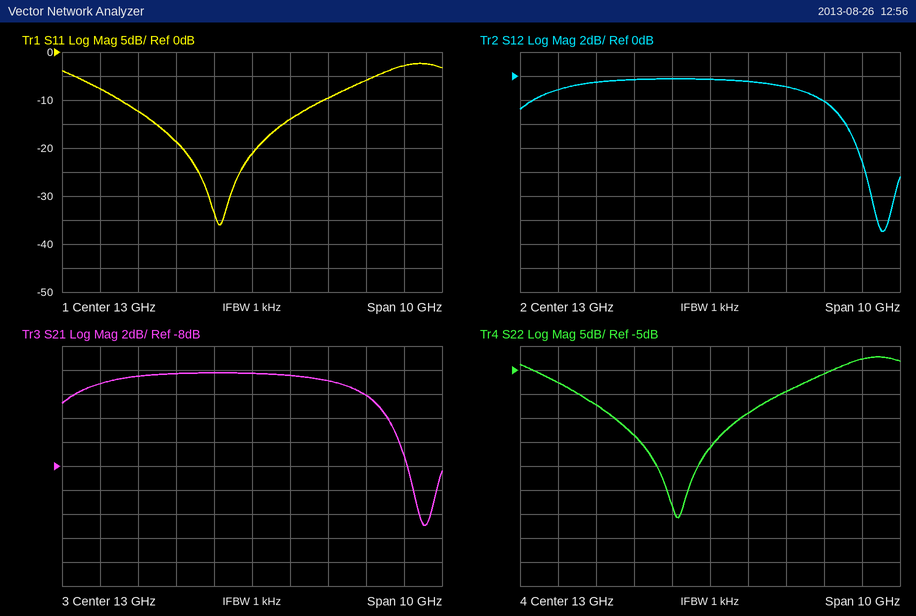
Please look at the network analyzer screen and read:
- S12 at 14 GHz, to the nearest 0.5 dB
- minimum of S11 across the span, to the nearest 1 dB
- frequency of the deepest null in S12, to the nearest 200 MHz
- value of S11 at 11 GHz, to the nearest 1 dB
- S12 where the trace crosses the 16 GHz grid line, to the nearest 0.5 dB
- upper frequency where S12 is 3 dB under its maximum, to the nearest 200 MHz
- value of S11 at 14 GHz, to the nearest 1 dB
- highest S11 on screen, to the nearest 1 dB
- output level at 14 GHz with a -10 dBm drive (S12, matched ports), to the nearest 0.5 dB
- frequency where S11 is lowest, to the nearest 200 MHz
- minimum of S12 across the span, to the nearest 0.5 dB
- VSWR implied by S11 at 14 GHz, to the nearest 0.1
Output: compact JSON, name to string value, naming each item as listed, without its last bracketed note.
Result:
{"S12 at 14 GHz, to the nearest 0.5 dB": "-0.5 dB", "minimum of S11 across the span, to the nearest 1 dB": "-36 dB", "frequency of the deepest null in S12, to the nearest 200 MHz": "17.6 GHz", "value of S11 at 11 GHz, to the nearest 1 dB": "-19 dB", "S12 where the trace crosses the 16 GHz grid line, to the nearest 0.5 dB": "-2.0 dB", "upper frequency where S12 is 3 dB under its maximum, to the nearest 200 MHz": "16.4 GHz", "value of S11 at 14 GHz, to the nearest 1 dB": "-14 dB", "highest S11 on screen, to the nearest 1 dB": "-2 dB", "output level at 14 GHz with a -10 dBm drive (S12, matched ports), to the nearest 0.5 dB": "-10.5 dBm", "frequency where S11 is lowest, to the nearest 200 MHz": "12.2 GHz", "minimum of S12 across the span, to the nearest 0.5 dB": "-13.0 dB", "VSWR implied by S11 at 14 GHz, to the nearest 0.1": "1.5"}
